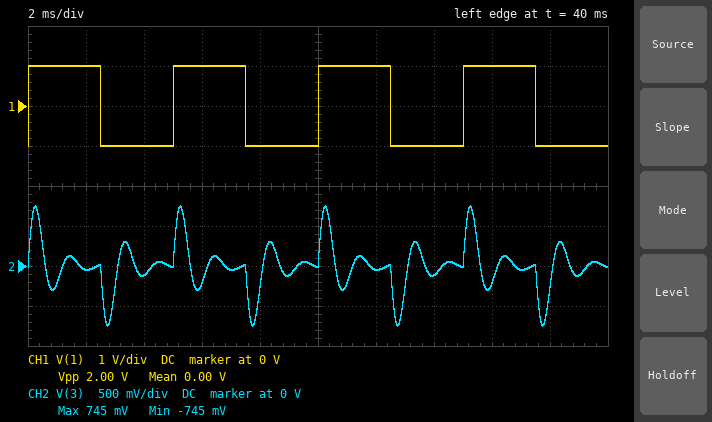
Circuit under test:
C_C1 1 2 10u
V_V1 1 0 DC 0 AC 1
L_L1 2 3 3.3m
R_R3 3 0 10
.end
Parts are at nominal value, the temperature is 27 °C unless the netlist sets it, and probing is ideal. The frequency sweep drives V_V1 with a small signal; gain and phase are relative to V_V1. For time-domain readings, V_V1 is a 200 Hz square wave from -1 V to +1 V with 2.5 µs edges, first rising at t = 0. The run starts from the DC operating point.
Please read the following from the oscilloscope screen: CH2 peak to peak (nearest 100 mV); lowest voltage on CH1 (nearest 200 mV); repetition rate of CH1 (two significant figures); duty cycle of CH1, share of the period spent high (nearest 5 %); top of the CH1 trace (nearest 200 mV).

1.5 V
-1.0 V
200 Hz
50 %
1.0 V
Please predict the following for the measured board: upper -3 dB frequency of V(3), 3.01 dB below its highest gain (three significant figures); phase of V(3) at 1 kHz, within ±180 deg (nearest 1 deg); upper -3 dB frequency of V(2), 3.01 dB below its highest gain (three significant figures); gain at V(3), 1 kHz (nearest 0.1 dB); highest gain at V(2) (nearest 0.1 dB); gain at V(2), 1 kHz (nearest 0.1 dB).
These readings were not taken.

1.15 kHz
-26 deg
1.41 kHz
-0.9 dB
6.5 dB
6.3 dB
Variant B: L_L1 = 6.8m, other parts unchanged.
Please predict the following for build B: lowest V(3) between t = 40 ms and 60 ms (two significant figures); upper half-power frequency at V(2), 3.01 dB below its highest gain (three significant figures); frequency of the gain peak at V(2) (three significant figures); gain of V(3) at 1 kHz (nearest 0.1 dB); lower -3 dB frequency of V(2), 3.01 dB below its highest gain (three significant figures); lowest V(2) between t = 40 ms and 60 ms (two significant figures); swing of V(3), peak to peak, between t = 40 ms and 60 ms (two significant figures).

-700 mV
810 Hz
631 Hz
-9.1 dB
531 Hz
-2.4 V
1.4 V
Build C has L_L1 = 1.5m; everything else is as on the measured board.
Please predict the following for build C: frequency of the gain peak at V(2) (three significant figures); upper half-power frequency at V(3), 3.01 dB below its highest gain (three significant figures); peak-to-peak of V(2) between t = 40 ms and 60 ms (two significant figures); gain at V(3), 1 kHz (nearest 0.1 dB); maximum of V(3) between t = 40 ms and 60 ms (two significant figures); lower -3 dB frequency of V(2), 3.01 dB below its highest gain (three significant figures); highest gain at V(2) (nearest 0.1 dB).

1.46 kHz
1.93 kHz
4.0 V
-1.5 dB
980 mV
1.00 kHz
4.3 dB
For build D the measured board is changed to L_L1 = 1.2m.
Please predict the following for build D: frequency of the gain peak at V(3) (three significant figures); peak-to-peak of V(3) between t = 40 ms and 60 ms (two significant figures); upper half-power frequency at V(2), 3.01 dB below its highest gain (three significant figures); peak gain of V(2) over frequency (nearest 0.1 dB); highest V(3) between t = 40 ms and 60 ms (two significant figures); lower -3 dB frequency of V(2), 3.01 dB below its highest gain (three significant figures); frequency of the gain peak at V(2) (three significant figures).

1.45 kHz
2.1 V
4.95 kHz
3.7 dB
1.0 V
1.09 kHz
1.67 kHz
